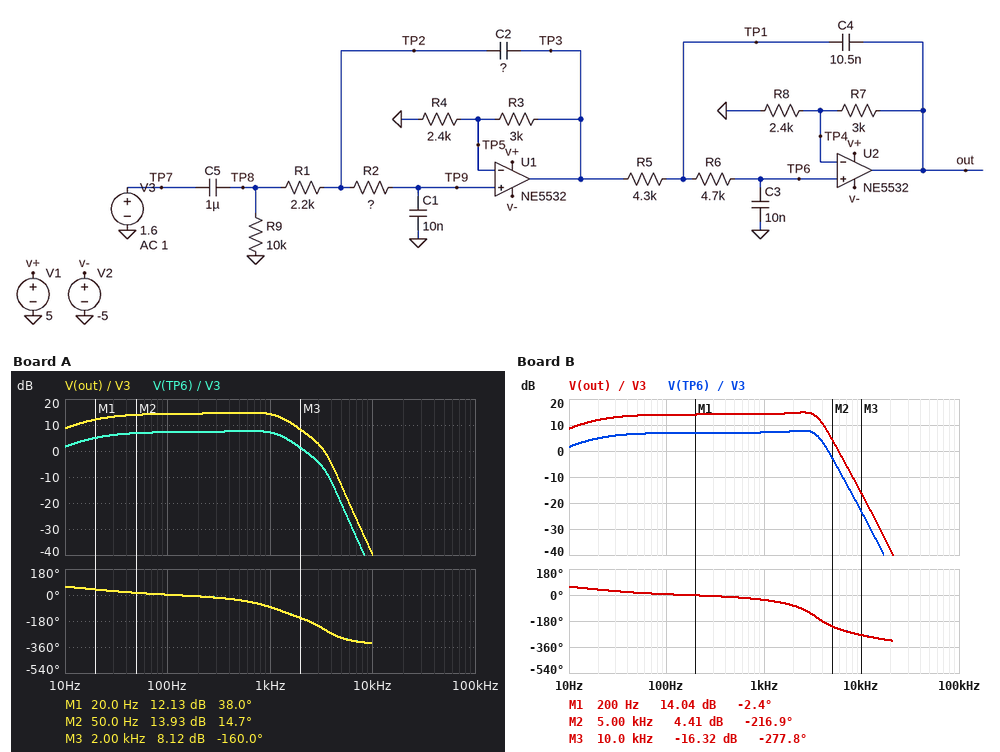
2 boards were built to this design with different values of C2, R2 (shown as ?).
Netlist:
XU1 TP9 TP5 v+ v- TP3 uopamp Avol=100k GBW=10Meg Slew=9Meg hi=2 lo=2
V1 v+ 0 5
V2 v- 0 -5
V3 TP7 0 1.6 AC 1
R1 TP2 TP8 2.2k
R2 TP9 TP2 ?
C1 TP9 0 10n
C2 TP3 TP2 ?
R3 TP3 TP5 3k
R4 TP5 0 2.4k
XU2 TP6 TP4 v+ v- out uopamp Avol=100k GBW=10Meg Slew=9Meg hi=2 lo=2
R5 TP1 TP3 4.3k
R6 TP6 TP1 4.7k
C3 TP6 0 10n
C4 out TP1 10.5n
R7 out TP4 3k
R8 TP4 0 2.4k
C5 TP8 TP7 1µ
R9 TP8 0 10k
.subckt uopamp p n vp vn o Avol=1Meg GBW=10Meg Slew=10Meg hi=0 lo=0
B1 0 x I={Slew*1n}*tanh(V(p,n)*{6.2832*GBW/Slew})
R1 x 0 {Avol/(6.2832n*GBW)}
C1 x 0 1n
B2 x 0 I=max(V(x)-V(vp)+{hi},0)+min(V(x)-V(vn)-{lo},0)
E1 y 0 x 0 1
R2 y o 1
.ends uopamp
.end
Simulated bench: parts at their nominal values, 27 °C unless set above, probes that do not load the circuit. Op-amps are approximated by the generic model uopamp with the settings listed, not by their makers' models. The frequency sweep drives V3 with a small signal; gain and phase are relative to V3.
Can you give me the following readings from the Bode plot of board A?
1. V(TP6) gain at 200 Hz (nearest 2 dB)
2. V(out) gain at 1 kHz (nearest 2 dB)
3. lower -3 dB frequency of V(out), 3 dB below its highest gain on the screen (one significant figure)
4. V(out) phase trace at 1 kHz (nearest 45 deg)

8 dB
14 dB
20 Hz
-90 deg
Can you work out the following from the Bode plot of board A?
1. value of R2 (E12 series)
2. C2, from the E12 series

22 kΩ
33 nF
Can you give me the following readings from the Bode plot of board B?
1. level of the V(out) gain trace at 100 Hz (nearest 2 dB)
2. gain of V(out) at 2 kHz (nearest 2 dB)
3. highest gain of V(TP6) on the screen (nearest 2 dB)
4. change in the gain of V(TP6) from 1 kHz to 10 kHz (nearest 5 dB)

14 dB
14 dB
8 dB
-30 dB
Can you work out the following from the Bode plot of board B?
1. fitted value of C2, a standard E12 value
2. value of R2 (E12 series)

5.6 nF
5.6 kΩ
